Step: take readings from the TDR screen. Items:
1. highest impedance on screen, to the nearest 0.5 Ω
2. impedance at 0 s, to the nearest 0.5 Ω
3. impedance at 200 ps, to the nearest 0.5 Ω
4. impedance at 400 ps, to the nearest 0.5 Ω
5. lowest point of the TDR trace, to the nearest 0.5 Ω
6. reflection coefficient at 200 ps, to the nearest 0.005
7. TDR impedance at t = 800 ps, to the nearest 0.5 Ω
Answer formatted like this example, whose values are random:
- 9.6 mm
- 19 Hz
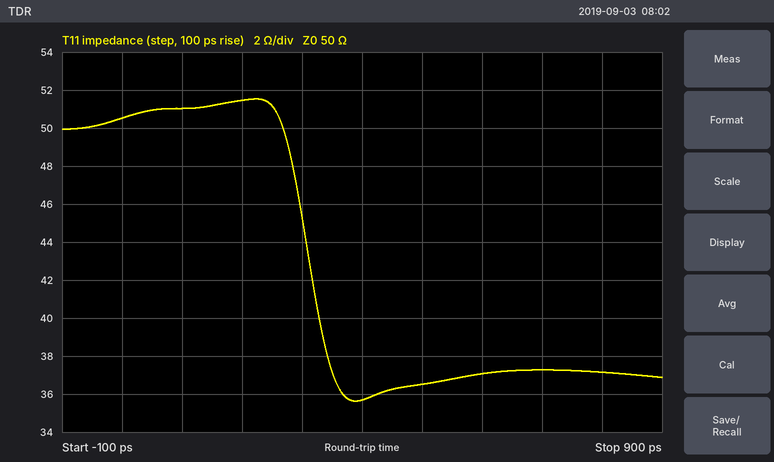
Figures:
- 51.5 Ω
- 50.5 Ω
- 51.5 Ω
- 35.5 Ω
- 35.5 Ω
- +0.015
- 37.0 Ω
